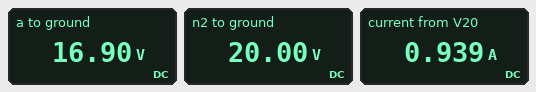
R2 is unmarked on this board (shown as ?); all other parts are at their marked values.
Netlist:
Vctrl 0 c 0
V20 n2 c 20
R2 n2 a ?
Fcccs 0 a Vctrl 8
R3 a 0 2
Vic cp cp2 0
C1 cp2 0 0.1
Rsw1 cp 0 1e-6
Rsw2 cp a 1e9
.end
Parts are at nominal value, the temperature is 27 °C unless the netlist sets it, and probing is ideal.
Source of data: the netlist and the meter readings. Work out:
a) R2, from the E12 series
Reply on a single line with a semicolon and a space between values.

3.3 Ω
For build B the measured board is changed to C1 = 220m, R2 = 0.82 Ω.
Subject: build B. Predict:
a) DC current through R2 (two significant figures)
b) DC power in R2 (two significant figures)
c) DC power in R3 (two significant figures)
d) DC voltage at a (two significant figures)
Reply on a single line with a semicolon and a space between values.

1.1 A; 930 mW; 180 W; 19 V
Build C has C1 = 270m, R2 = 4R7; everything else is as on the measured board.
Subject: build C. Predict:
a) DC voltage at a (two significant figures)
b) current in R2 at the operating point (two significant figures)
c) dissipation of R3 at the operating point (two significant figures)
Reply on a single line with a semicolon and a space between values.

16 V; 880 mA; 130 W
